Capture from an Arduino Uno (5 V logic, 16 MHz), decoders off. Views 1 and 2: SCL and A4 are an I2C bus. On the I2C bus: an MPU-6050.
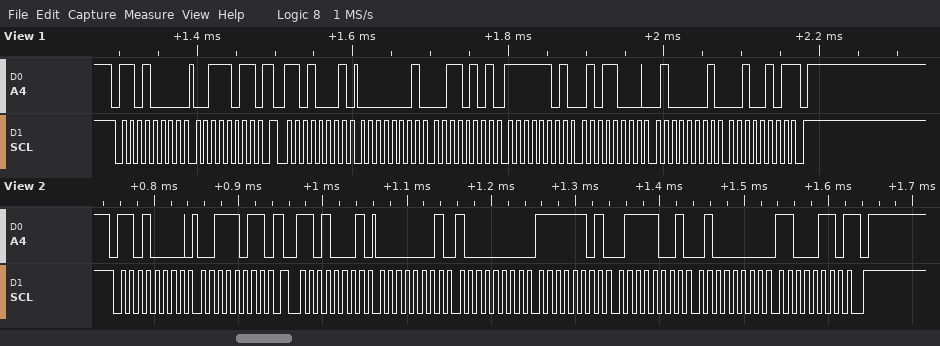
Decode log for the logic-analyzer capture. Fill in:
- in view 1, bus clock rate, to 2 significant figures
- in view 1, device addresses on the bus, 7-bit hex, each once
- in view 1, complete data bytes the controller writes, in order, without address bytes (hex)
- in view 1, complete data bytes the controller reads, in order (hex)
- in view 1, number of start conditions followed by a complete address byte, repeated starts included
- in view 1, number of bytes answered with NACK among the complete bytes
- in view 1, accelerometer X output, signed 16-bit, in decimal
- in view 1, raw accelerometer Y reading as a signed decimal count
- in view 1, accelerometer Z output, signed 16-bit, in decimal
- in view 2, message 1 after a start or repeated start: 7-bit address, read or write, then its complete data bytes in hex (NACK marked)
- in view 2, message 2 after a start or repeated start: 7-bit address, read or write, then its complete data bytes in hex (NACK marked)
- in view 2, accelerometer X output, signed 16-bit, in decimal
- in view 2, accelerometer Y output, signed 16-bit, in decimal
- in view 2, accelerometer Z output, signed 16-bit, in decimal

100 kHz
0x68
3B
01 35 FD 58 41 25
2
1
309
-680
16677
0x68 write: 3B
0x68 read: 01 80 FD 79 40 C6 NACK
384
-647
16582
